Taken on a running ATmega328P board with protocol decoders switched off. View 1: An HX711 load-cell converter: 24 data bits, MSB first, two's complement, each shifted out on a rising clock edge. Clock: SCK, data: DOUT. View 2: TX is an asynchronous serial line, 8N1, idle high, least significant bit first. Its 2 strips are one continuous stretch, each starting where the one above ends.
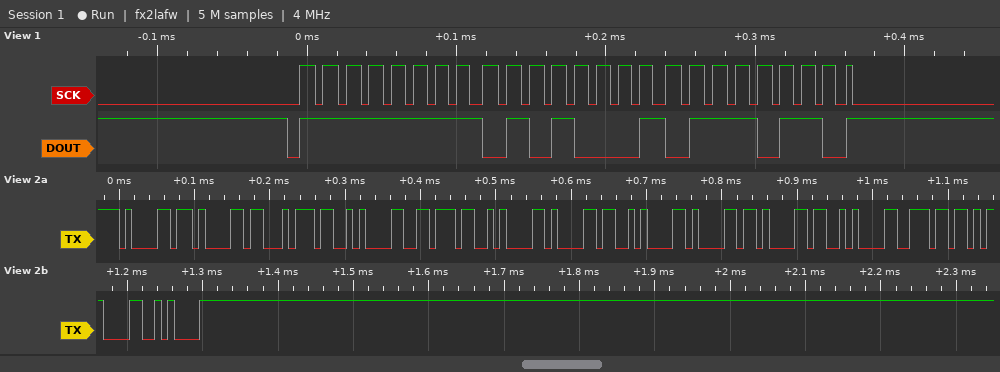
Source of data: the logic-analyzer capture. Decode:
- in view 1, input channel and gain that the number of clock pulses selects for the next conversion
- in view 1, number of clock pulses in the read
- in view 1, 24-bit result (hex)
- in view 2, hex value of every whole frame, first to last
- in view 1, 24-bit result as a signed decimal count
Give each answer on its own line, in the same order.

channel A, gain 128
25
0xFF5176
61 61 74 0A 76 0A 61 0A 61 61 0A 6E 0D 0A
-44682
